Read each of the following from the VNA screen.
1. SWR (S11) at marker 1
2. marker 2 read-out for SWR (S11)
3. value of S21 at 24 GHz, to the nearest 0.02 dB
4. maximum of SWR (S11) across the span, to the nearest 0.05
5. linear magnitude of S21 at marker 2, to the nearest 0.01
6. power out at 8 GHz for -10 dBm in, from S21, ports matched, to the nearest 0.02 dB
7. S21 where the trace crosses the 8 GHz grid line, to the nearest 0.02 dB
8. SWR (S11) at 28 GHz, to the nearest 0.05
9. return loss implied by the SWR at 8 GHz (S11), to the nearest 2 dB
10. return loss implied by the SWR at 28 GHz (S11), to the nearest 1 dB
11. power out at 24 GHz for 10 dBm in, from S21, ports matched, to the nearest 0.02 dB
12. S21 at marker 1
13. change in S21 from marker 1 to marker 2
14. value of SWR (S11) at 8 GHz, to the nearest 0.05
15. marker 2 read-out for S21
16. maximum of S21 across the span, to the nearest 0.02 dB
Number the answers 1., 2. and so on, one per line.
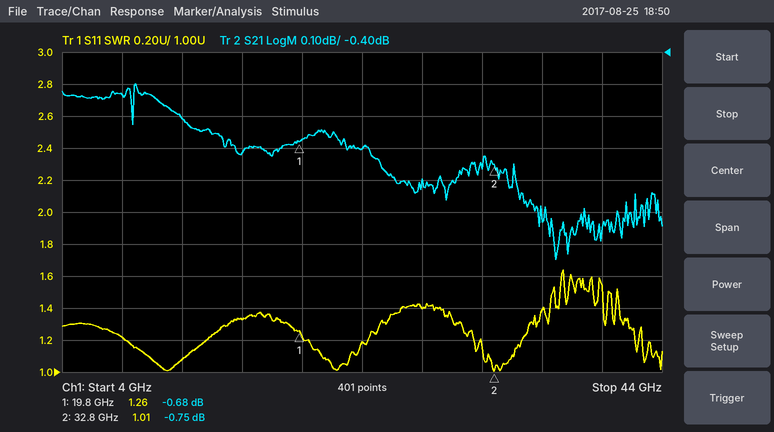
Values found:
1. 1.26
2. 1.01
3. -0.70 dB
4. 1.65
5. 0.92
6. -10.54 dBm
7. -0.54 dB
8. 1.40
9. 20 dB
10. 16 dB
11. 9.30 dBm
12. -0.68 dB
13. -0.07 dB
14. 1.20
15. -0.75 dB
16. -0.50 dB
